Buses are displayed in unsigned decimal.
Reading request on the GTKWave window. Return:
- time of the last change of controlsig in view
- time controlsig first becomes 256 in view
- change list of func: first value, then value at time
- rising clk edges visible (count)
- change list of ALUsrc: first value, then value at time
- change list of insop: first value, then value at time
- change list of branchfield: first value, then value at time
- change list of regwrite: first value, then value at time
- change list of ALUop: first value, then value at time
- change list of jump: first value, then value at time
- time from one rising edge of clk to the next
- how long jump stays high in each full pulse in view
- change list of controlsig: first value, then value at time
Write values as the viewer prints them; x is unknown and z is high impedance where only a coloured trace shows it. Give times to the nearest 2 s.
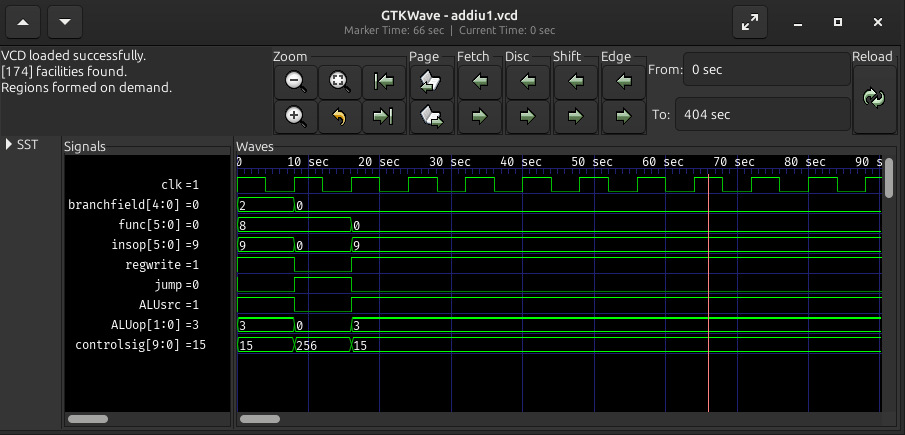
16 s
8 s
8, 0 at 16 s
11
1, 0 at 8 s, 1 at 16 s
9, 0 at 8 s, 9 at 16 s
2, 0 at 8 s
1, 0 at 8 s, 1 at 16 s
3, 0 at 8 s, 3 at 16 s
0, 1 at 8 s, 0 at 16 s
8 s
8 s
15, 256 at 8 s, 15 at 16 s
